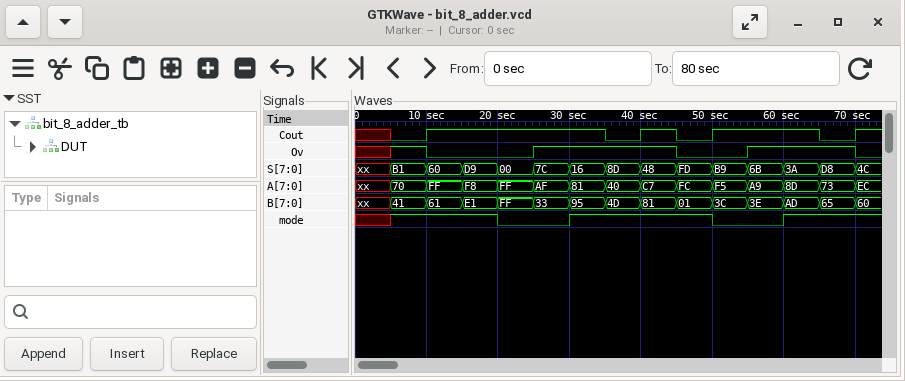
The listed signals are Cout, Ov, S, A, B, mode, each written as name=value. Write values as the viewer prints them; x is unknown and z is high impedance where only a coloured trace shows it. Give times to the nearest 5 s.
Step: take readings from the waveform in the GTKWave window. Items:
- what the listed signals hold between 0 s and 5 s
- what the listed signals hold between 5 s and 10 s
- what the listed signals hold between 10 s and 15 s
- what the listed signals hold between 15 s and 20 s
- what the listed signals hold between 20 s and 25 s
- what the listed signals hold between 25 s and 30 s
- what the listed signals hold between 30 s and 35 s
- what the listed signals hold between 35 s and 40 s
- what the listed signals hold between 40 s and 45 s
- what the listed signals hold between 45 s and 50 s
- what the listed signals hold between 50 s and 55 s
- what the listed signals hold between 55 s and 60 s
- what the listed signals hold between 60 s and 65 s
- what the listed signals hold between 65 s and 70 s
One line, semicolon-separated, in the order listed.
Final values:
Cout=x, Ov=x, S=xx, A=xx, B=xx, mode=x; Cout=0, Ov=1, S=B1, A=70, B=41, mode=1; Cout=1, Ov=0, S=60, A=FF, B=61, mode=1; Cout=1, Ov=0, S=D9, A=F8, B=E1, mode=1; Cout=1, Ov=0, S=00, A=FF, B=FF, mode=0; Cout=1, Ov=1, S=7C, A=AF, B=33, mode=0; Cout=1, Ov=1, S=16, A=81, B=95, mode=1; Cout=0, Ov=1, S=8D, A=40, B=4D, mode=1; Cout=1, Ov=1, S=48, A=C7, B=81, mode=1; Cout=0, Ov=0, S=FD, A=FC, B=01, mode=1; Cout=1, Ov=0, S=B9, A=F5, B=3C, mode=0; Cout=1, Ov=1, S=6B, A=A9, B=3E, mode=0; Cout=1, Ov=1, S=3A, A=8D, B=AD, mode=1; Cout=0, Ov=1, S=D8, A=73, B=65, mode=1
